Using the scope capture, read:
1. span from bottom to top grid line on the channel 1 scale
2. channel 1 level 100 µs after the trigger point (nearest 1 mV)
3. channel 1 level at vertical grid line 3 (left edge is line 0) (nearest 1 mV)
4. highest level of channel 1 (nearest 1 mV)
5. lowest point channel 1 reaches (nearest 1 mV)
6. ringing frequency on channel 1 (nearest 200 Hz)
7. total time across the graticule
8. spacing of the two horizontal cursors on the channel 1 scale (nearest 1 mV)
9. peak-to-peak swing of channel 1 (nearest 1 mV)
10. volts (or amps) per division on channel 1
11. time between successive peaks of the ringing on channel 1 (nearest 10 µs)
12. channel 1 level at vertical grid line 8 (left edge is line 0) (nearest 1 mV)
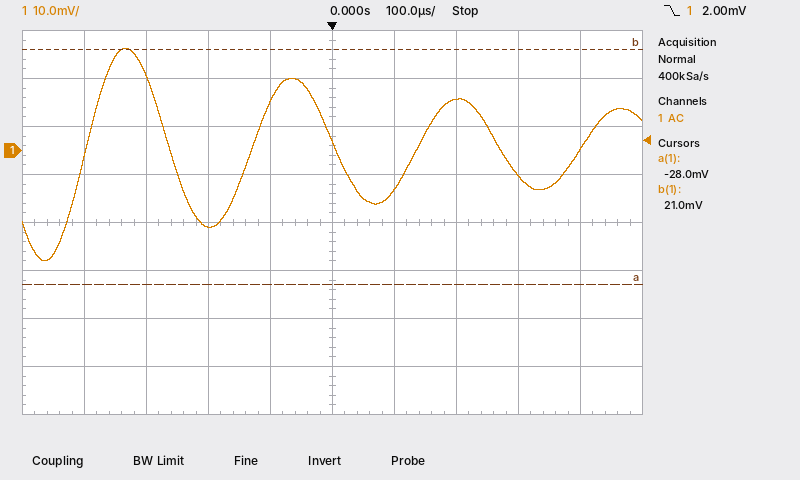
80 mV
-8 mV
-16 mV
21 mV
-23 mV
3.8 kHz
1 ms
49 mV
44 mV
10 mV
270 µs
-5 mV
